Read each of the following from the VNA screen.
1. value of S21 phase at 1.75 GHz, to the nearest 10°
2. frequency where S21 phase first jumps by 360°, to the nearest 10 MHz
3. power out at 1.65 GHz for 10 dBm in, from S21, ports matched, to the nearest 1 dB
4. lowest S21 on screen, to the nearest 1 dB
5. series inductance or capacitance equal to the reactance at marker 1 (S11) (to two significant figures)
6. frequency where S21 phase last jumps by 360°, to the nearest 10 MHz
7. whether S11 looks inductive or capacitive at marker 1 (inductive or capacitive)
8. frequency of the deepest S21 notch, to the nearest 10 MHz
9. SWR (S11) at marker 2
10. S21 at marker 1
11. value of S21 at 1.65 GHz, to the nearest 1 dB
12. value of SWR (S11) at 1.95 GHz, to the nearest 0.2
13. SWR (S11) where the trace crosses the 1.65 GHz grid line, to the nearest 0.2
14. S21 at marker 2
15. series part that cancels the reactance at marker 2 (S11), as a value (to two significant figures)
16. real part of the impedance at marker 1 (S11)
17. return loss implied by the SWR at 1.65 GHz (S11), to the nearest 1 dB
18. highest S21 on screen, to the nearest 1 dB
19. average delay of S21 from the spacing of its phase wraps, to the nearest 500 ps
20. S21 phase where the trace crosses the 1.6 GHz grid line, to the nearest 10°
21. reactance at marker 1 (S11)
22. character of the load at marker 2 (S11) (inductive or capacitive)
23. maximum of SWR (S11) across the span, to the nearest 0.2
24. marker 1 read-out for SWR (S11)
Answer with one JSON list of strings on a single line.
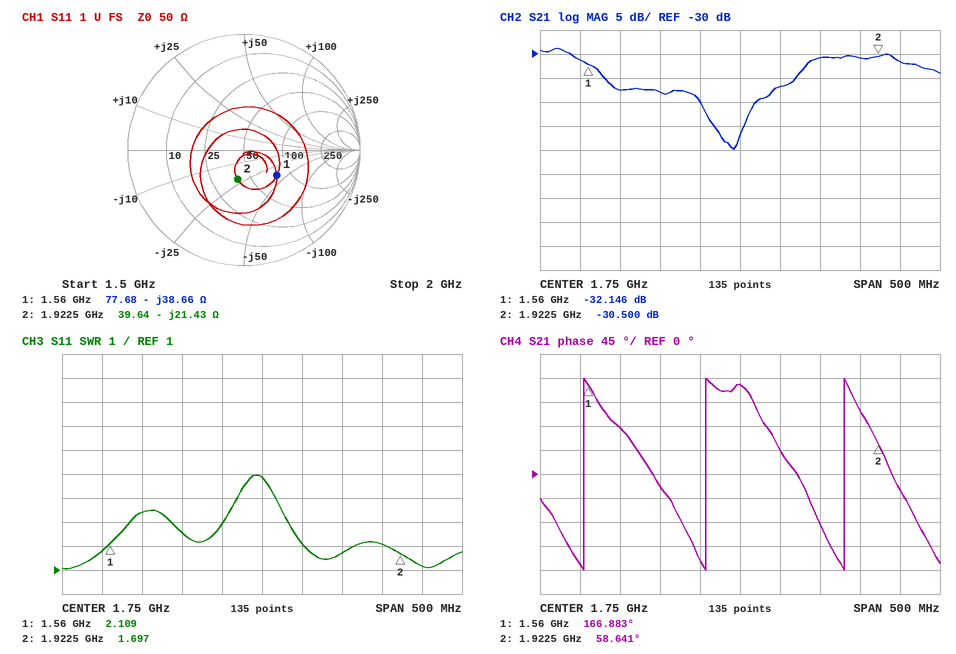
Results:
["170°", "1.55 GHz", "-28 dBm", "-50 dB", "2.6 pF", "1.88 GHz", "capacitive", "1.74 GHz", "1.697", "-32.146 dB", "-38 dB", "1.2", "2.6", "-30.500 dB", "1.8 nH", "77.68 Ω", "7 dB", "-29 dB", "6.0 ns", "90°", "-38.66 Ω", "capacitive", "5.0", "2.109"]
